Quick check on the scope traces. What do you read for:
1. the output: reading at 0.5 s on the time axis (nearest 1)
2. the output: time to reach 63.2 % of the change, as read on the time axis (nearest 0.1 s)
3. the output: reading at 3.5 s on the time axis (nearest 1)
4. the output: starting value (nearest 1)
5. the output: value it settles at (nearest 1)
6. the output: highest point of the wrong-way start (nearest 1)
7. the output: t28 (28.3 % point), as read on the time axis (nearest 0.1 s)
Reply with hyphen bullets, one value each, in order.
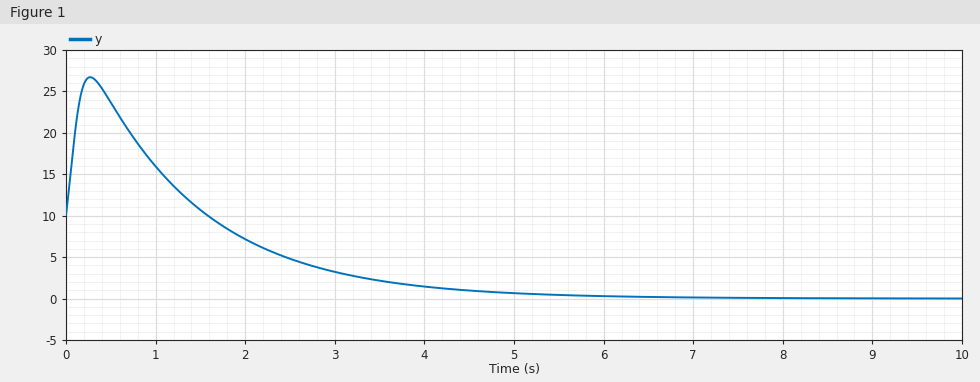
- 24
- 2.8 s
- 2
- 10
- 0
- 27
- 2.0 s
